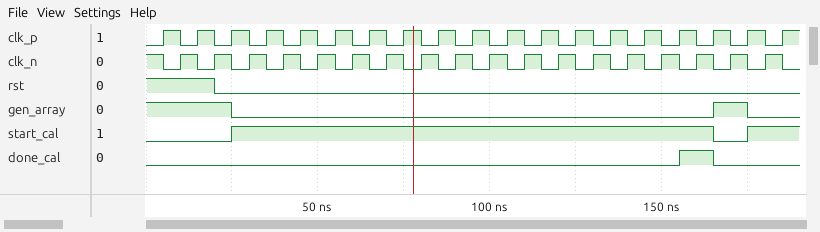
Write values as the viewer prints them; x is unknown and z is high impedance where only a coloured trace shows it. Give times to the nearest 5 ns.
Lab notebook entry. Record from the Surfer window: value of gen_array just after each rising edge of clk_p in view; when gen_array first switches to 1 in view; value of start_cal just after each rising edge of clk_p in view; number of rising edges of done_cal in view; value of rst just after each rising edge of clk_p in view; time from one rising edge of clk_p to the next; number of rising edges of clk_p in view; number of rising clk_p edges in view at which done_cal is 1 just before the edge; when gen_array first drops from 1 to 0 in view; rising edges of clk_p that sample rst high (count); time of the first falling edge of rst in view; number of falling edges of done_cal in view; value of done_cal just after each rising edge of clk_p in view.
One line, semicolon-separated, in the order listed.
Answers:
1 1 0 0 0 0 0 0 0 0 0 0 0 0 0 0 1 0 0; 165 ns; 0 0 1 1 1 1 1 1 1 1 1 1 1 1 1 1 0 1 1; 1; 1 1 0 0 0 0 0 0 0 0 0 0 0 0 0 0 0 0 0; 10 ns; 19; 1; 25 ns; 2; 20 ns; 1; 0 0 0 0 0 0 0 0 0 0 0 0 0 0 0 1 0 0 0
